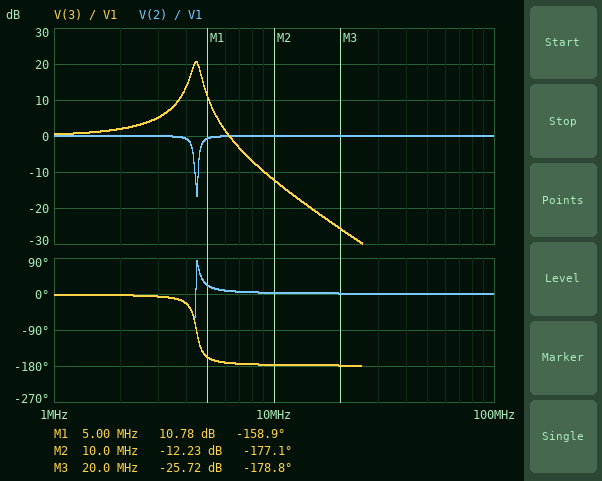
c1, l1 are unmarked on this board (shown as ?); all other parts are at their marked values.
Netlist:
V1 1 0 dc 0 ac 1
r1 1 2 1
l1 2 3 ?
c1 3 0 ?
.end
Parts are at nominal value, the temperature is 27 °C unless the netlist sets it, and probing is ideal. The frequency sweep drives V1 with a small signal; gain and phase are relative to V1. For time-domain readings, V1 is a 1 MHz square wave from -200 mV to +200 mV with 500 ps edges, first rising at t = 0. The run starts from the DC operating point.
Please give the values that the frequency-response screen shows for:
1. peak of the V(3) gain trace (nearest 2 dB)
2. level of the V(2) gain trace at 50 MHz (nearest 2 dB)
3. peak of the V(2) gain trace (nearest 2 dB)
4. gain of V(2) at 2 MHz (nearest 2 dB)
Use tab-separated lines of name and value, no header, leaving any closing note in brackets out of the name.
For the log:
peak of the V(3) gain trace	20 dB
level of the V(2) gain trace at 50 MHz	0 dB
peak of the V(2) gain trace	0 dB
gain of V(2) at 2 MHz	0 dB
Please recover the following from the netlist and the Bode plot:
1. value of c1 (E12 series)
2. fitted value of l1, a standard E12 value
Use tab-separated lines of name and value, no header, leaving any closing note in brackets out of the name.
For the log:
value of c1	3.3 nF
fitted value of l1, a standard E12 value	390 nH
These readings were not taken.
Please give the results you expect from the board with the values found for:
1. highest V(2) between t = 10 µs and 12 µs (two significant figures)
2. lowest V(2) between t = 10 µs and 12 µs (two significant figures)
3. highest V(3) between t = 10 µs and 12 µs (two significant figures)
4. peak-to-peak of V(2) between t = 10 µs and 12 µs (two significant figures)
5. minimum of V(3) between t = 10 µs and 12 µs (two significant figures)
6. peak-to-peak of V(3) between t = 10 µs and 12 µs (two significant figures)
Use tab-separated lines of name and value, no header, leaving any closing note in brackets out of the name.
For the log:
highest V(2) between t = 10 µs and 12 µs	220 mV
lowest V(2) between t = 10 µs and 12 µs	-220 mV
highest V(3) between t = 10 µs and 12 µs	480 mV
peak-to-peak of V(2) between t = 10 µs and 12 µs	450 mV
minimum of V(3) between t = 10 µs and 12 µs	-480 mV
peak-to-peak of V(3) between t = 10 µs and 12 µs	950 mV
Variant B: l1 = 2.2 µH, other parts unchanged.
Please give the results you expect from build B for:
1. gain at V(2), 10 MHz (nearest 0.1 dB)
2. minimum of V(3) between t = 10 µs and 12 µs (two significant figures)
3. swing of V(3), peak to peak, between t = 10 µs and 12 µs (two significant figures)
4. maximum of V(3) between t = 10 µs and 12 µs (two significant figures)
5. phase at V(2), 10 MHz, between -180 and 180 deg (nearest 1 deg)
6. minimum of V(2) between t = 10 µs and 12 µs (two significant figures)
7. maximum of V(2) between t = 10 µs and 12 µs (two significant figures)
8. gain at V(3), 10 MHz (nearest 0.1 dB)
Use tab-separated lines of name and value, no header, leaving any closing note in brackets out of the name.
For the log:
gain at V(2), 10 MHz	0 dB
minimum of V(3) between t = 10 µs and 12 µs	-420 mV
swing of V(3), peak to peak, between t = 10 µs and 12 µs	810 mV
maximum of V(3) between t = 10 µs and 12 µs	390 mV
phase at V(2), 10 MHz, between -180 and 180 deg	0 deg
minimum of V(2) between t = 10 µs and 12 µs	-210 mV
maximum of V(2) between t = 10 µs and 12 µs	210 mV
gain at V(3), 10 MHz	-28.8 dB
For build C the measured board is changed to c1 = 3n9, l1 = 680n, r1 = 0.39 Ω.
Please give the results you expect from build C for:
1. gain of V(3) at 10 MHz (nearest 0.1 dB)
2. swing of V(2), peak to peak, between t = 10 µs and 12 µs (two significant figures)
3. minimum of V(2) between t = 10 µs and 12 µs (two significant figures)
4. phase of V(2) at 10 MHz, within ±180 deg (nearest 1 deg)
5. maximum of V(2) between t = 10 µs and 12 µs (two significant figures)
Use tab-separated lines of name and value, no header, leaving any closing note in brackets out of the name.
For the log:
gain of V(3) at 10 MHz	-19.5 dB
swing of V(2), peak to peak, between t = 10 µs and 12 µs	470 mV
minimum of V(2) between t = 10 µs and 12 µs	-240 mV
phase of V(2) at 10 MHz, within ±180 deg	1 deg
maximum of V(2) between t = 10 µs and 12 µs	240 mV
